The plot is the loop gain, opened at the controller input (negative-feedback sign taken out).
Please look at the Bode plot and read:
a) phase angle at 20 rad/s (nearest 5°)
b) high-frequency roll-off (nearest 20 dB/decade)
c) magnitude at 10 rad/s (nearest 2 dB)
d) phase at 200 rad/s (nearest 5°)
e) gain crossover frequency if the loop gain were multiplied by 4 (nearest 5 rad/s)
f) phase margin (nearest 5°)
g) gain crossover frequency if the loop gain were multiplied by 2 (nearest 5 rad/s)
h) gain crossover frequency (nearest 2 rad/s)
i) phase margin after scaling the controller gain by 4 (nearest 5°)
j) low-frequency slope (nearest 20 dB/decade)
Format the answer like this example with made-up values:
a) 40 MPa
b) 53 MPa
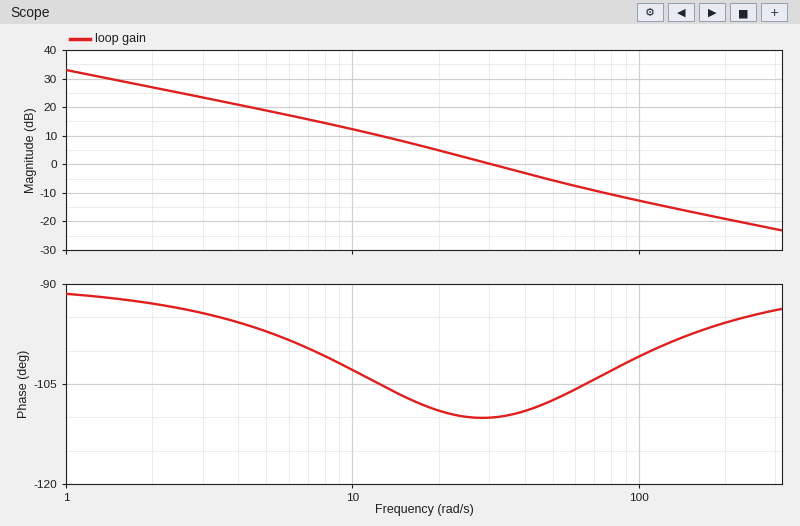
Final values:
a) -110°
b) -20 dB/decade
c) 12 dB
d) -95°
e) 95 rad/s
f) 70°
g) 50 rad/s
h) 30 rad/s
i) 80°
j) -20 dB/decade
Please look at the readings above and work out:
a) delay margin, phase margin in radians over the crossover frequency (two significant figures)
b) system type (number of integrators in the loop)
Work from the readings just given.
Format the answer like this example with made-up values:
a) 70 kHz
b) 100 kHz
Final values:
a) 0.041 s
b) 1
